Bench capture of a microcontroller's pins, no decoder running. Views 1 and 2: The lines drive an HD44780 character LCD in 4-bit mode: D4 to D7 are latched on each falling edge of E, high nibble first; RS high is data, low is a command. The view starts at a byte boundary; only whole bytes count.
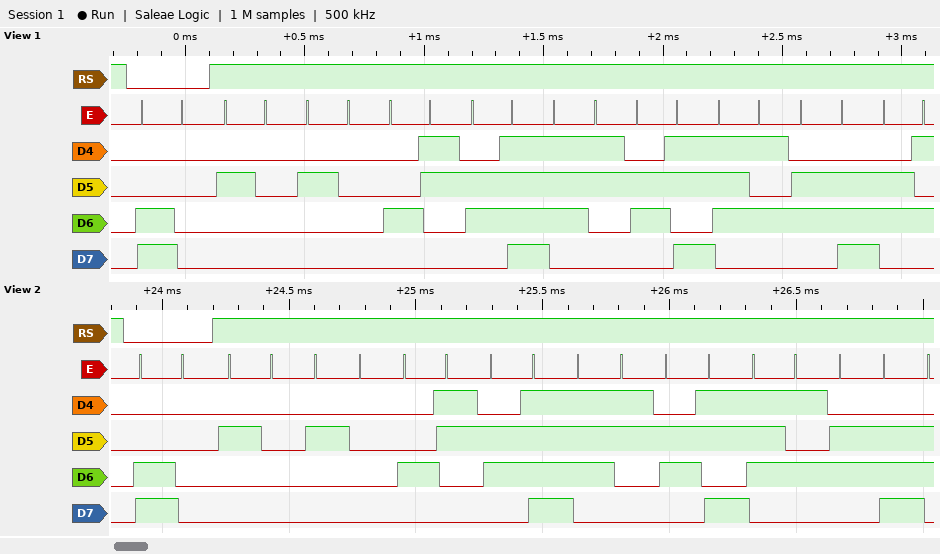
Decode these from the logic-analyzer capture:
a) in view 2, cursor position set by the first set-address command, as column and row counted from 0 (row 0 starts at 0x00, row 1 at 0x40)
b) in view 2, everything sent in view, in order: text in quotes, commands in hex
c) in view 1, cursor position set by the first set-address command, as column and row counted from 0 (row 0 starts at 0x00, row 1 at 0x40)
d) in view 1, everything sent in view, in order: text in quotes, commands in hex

column 0, row 1
0xC0 "  Coskun"
column 0, row 1
0xC0 "  Coskune"
